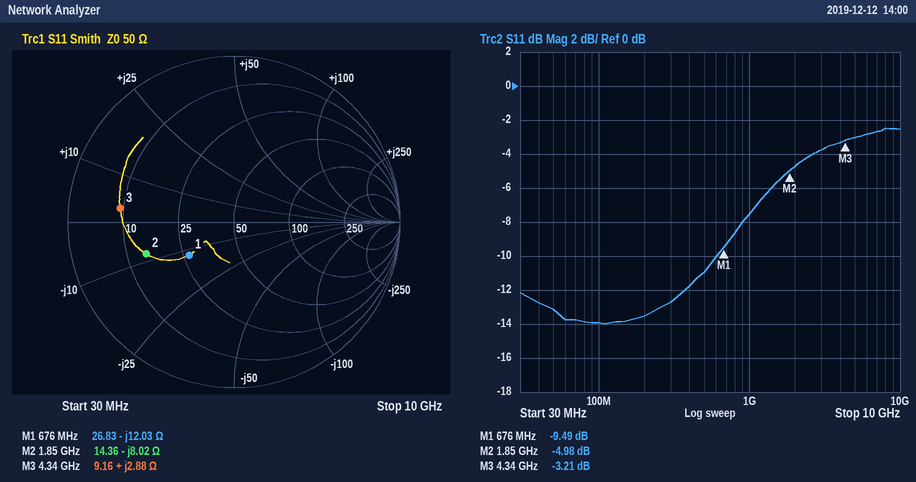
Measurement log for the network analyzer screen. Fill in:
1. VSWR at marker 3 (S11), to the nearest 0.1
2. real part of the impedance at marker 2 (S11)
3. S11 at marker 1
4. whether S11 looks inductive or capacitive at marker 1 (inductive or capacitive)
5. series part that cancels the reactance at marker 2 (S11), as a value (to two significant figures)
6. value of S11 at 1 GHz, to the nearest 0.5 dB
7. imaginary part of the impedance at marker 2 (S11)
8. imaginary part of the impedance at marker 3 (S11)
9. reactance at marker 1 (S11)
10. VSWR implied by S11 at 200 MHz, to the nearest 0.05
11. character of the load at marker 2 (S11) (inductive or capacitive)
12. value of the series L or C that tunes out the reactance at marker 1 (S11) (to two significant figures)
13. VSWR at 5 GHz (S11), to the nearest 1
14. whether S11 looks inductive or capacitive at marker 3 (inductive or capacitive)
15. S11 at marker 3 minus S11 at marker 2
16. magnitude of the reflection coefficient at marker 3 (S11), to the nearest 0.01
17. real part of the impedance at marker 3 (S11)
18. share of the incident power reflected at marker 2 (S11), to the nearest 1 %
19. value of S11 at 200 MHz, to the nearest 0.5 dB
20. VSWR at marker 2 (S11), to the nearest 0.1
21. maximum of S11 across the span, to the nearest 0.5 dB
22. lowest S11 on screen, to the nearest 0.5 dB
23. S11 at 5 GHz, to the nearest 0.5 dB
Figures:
5.5
14.36 Ω
-9.49 dB
capacitive
690 pH
-7.5 dB
-8.02 Ω
+2.88 Ω
-12.03 Ω
1.55
capacitive
2.8 nH
6
inductive
1.77 dB
0.69
9.16 Ω
32 %
-13.5 dB
3.6
-2.5 dB
-14.0 dB
-3.0 dB
